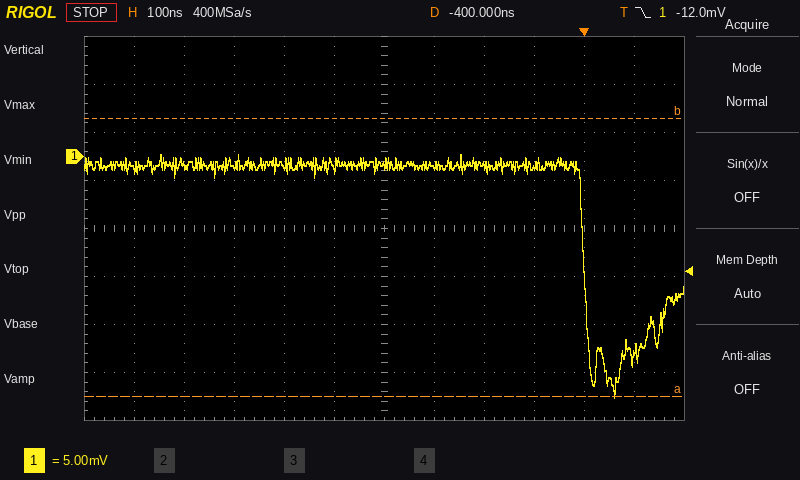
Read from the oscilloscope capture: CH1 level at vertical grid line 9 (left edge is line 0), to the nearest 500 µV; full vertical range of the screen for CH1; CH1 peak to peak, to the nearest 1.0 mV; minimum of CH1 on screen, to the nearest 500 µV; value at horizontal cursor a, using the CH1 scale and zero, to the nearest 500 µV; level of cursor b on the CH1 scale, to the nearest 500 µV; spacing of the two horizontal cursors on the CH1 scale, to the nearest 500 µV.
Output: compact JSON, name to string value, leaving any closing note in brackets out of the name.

{"CH1 level at vertical grid line 9 (left edge is line 0), to the nearest 500 µV": "-1.0 mV", "full vertical range of the screen for CH1": "40 mV", "CH1 peak to peak, to the nearest 1.0 mV": "25.0 mV", "minimum of CH1 on screen, to the nearest 500 µV": "-25.0 mV", "value at horizontal cursor a, using the CH1 scale and zero, to the nearest 500 µV": "-25.0 mV", "level of cursor b on the CH1 scale, to the nearest 500 µV": "4.0 mV", "spacing of the two horizontal cursors on the CH1 scale, to the nearest 500 µV": "29.0 mV"}
